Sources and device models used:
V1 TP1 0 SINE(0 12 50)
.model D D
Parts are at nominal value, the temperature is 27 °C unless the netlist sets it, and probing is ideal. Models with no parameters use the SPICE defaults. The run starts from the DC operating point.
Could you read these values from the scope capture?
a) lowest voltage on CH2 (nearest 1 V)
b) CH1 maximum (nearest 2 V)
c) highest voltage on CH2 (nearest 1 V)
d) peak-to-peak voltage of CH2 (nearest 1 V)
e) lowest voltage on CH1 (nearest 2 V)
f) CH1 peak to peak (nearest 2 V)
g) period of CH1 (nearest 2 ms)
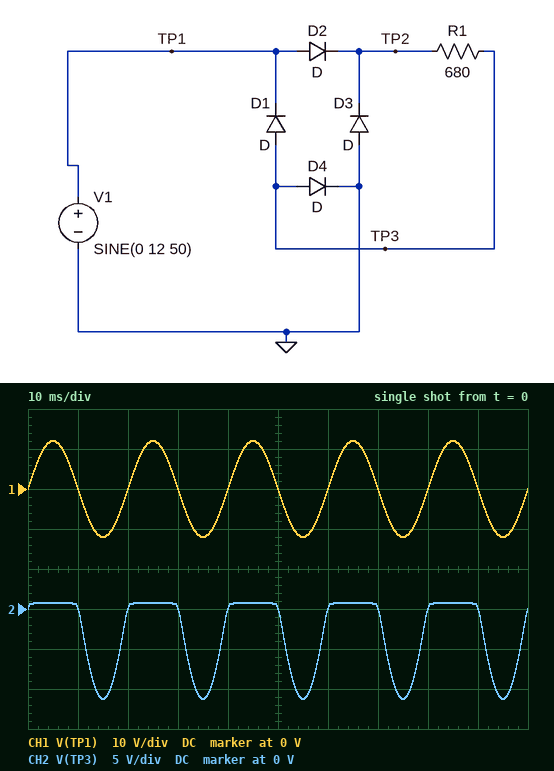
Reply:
-11 V
12 V
1 V
12 V
-12 V
24 V
20 ms
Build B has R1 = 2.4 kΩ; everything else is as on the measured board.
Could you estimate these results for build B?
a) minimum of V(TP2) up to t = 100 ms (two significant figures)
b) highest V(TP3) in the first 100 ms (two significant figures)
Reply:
-690 mV
690 mV
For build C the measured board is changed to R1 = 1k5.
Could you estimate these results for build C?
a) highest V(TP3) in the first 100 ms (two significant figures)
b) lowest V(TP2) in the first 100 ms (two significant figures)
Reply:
710 mV
-710 mV
